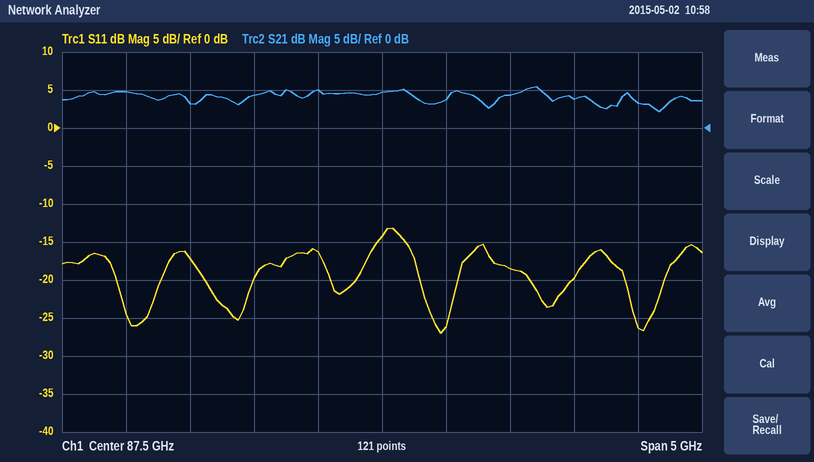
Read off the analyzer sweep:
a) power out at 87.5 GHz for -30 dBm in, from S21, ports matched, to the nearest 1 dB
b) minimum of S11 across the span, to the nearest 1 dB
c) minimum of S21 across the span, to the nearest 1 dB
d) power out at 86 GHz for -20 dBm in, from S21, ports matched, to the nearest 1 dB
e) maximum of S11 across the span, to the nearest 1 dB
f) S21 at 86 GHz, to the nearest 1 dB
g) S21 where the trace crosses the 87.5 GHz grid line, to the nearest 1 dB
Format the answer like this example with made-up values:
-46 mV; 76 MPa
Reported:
-25 dBm; -27 dB; 2 dB; -17 dBm; -13 dB; 3 dB; 5 dB
